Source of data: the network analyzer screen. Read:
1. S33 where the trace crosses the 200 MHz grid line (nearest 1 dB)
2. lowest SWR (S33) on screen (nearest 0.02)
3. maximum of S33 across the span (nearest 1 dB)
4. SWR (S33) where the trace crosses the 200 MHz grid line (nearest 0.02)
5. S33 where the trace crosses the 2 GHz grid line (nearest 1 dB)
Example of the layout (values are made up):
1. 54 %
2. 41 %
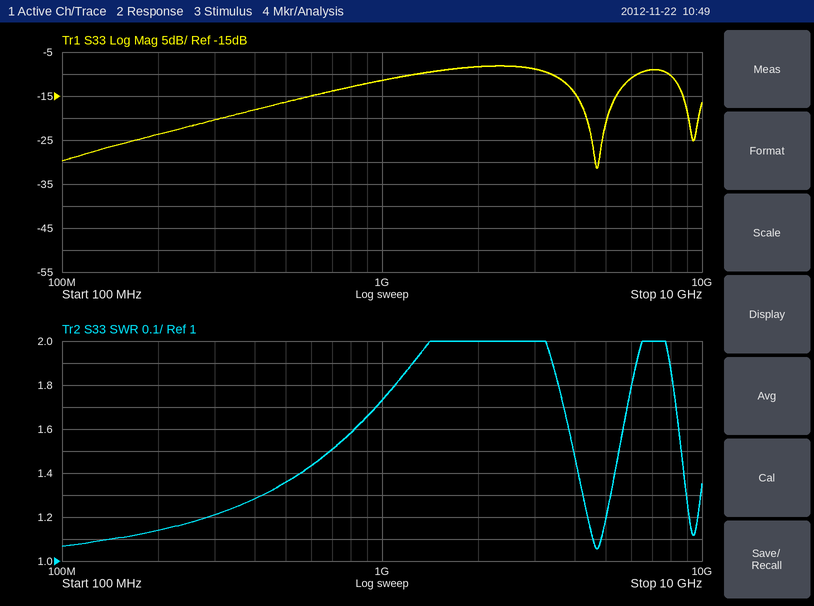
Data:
1. -24 dB
2. 1.06
3. -8 dB
4. 1.14
5. -8 dB
